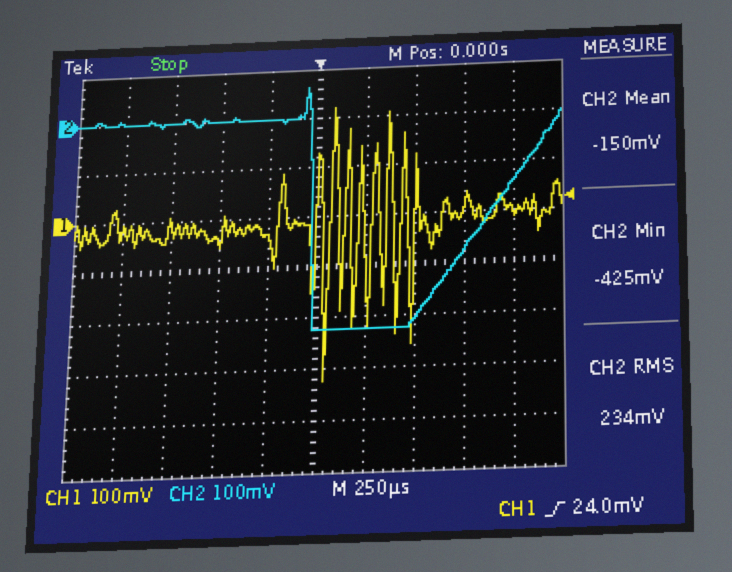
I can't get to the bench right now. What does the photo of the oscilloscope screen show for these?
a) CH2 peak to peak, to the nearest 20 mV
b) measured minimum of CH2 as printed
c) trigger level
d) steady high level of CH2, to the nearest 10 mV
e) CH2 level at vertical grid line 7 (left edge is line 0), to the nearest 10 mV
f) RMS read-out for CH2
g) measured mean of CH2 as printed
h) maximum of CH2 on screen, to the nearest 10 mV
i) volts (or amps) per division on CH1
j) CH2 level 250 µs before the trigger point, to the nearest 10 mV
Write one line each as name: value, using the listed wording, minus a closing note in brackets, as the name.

CH2 peak to peak, to the nearest 20 mV: 480 mV
measured minimum of CH2 as printed: -425 mV
trigger level: 24.0 mV
steady high level of CH2, to the nearest 10 mV: 0 mV
CH2 level at vertical grid line 7 (left edge is line 0), to the nearest 10 mV: -410 mV
RMS read-out for CH2: 234 mV
measured mean of CH2 as printed: -150 mV
maximum of CH2 on screen, to the nearest 10 mV: 60 mV
volts (or amps) per division on CH1: 100 mV
CH2 level 250 µs before the trigger point, to the nearest 10 mV: 0 mV
